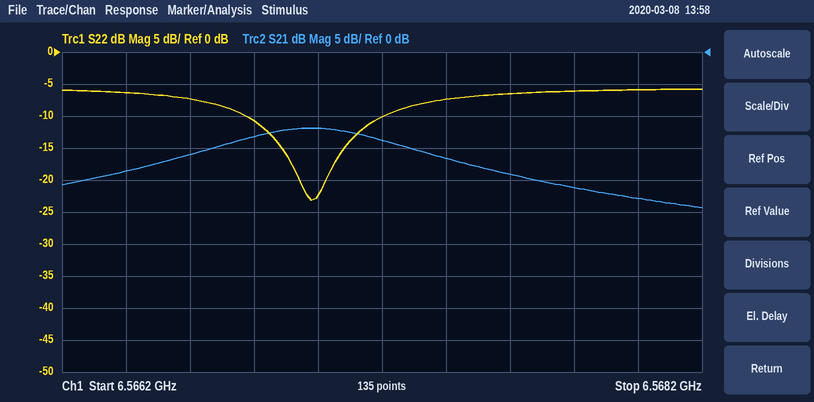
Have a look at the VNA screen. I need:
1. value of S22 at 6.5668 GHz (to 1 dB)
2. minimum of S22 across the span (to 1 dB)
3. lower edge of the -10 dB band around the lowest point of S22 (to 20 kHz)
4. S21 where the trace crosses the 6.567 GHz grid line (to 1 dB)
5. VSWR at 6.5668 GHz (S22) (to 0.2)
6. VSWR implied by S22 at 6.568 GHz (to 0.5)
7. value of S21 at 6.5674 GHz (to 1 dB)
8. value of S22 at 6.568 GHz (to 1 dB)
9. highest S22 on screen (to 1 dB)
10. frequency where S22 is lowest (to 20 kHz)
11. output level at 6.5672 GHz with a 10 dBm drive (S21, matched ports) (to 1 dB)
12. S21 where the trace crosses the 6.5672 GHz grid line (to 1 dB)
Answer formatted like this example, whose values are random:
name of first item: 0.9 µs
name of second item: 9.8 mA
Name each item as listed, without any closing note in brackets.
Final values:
value of S22 at 6.5668 GHz: -11 dB
minimum of S22 across the span: -23 dB
lower edge of the -10 dB band around the lowest point of S22: 6.56678 GHz
S21 where the trace crosses the 6.567 GHz grid line: -12 dB
VSWR at 6.5668 GHz (S22): 1.8
VSWR implied by S22 at 6.568 GHz: 3.0
value of S21 at 6.5674 GHz: -17 dB
value of S22 at 6.568 GHz: -6 dB
highest S22 on screen: -6 dB
frequency where S22 is lowest: 6.56698 GHz
output level at 6.5672 GHz with a 10 dBm drive (S21, matched ports): -4 dBm
S21 where the trace crosses the 6.5672 GHz grid line: -14 dB
